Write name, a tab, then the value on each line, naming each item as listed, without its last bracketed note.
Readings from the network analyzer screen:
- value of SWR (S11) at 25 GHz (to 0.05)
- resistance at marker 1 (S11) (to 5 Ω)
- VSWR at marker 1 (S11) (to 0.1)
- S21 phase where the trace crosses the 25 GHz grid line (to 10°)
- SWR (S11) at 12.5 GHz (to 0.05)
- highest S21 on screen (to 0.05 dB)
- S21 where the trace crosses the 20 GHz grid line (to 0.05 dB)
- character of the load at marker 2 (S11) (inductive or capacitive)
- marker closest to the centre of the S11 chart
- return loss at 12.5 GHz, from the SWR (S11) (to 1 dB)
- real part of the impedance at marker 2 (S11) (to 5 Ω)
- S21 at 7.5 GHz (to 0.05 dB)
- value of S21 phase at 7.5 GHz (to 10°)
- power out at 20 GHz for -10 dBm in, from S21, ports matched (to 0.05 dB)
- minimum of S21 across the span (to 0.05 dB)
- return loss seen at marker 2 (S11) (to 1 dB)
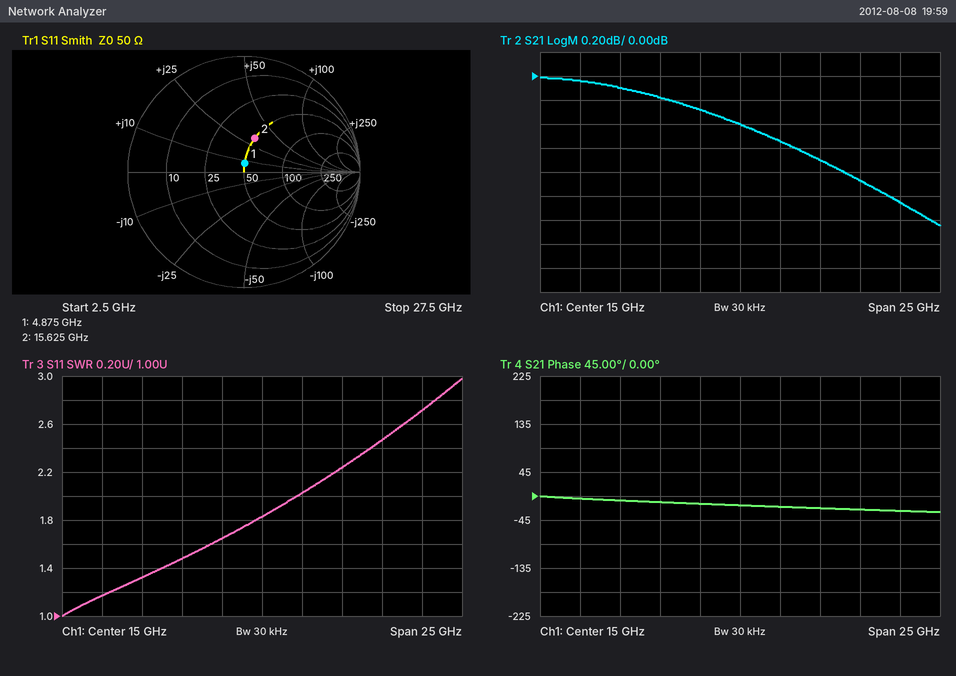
value of SWR (S11) at 25 GHz	2.70
resistance at marker 1 (S11)	50 Ω
VSWR at marker 1 (S11)	1.2
S21 phase where the trace crosses the 25 GHz grid line	-30°
SWR (S11) at 12.5 GHz	1.65
highest S21 on screen	0.00 dB
S21 where the trace crosses the 20 GHz grid line	-0.70 dB
character of the load at marker 2 (S11)	inductive
marker closest to the centre of the S11 chart	marker 1
return loss at 12.5 GHz, from the SWR (S11)	12 dB
real part of the impedance at marker 2 (S11)	50 Ω
S21 at 7.5 GHz	-0.10 dB
value of S21 phase at 7.5 GHz	-10°
power out at 20 GHz for -10 dBm in, from S21, ports matched	-10.70 dBm
minimum of S21 across the span	-1.25 dB
return loss seen at marker 2 (S11)	10 dB
